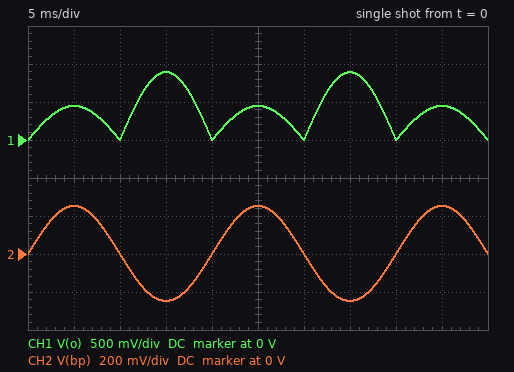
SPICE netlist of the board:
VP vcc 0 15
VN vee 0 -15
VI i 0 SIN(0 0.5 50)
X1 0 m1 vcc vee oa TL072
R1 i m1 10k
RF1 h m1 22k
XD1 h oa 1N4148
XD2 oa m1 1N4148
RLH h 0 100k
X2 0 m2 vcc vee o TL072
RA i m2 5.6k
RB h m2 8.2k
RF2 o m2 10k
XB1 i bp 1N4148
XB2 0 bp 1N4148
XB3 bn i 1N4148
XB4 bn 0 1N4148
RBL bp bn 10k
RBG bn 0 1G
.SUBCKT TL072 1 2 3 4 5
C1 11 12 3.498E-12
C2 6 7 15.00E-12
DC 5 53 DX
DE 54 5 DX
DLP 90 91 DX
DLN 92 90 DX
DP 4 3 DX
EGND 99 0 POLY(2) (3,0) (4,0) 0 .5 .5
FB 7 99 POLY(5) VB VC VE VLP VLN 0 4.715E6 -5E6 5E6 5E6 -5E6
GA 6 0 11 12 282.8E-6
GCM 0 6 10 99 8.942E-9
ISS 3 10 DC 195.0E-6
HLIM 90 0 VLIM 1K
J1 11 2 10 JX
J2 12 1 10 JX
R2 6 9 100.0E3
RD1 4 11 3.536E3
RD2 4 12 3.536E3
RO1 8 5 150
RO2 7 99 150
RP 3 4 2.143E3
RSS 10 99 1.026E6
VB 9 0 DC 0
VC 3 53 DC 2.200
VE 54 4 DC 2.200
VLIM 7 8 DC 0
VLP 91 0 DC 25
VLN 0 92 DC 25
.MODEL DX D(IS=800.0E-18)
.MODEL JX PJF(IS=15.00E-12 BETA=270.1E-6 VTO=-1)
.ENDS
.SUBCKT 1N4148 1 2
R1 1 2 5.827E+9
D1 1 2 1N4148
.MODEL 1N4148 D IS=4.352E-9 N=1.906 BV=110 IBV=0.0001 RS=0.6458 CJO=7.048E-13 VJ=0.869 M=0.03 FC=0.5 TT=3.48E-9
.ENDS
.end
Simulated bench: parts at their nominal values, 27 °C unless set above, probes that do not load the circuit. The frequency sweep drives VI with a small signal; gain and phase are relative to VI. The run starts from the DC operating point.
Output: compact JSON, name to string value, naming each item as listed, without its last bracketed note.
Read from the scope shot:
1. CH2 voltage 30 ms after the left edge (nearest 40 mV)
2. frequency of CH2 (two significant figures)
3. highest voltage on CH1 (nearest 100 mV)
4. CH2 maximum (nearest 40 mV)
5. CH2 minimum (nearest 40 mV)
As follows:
{"CH2 voltage 30 ms after the left edge": "0 V", "frequency of CH2": "50 Hz", "highest voltage on CH1": "900 mV", "CH2 maximum": "240 mV", "CH2 minimum": "-240 mV"}
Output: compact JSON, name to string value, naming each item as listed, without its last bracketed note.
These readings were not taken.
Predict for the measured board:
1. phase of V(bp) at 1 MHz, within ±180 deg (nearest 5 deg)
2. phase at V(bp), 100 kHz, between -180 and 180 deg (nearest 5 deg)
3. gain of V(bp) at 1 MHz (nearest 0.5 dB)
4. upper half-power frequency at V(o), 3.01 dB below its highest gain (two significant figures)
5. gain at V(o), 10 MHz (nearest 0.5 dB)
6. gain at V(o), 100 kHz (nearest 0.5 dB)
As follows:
{"phase of V(bp) at 1 MHz, within ±180 deg": "0 deg", "phase at V(bp), 100 kHz, between -180 and 180 deg": "0 deg", "gain of V(bp) at 1 MHz": "-6.0 dB", "upper half-power frequency at V(o), 3.01 dB below its highest gain": "1.3 MHz", "gain at V(o), 10 MHz": "-18.0 dB", "gain at V(o), 100 kHz": "5.5 dB"}
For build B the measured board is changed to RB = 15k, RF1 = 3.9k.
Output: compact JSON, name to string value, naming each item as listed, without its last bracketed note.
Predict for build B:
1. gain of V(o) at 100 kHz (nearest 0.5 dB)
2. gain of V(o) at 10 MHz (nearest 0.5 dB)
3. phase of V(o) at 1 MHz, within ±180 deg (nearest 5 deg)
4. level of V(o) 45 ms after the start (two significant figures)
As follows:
{"gain of V(o) at 100 kHz": "6.0 dB", "gain of V(o) at 10 MHz": "-17.5 dB", "phase of V(o) at 1 MHz, within ±180 deg": "130 deg", "level of V(o) 45 ms after the start": "-760 mV"}
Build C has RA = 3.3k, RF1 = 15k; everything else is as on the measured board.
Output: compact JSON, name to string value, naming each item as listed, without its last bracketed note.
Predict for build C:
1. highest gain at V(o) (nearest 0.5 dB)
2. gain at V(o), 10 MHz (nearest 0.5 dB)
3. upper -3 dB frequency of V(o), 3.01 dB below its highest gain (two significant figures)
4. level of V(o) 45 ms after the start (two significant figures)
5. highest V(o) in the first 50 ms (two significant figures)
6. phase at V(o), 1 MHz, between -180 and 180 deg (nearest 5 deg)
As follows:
{"highest gain at V(o)": "10.0 dB", "gain at V(o), 10 MHz": "-16.5 dB", "upper -3 dB frequency of V(o), 3.01 dB below its highest gain": "880 kHz", "level of V(o) 45 ms after the start": "-600 mV", "highest V(o) in the first 50 ms": "1.5 V", "phase at V(o), 1 MHz, between -180 and 180 deg": "120 deg"}
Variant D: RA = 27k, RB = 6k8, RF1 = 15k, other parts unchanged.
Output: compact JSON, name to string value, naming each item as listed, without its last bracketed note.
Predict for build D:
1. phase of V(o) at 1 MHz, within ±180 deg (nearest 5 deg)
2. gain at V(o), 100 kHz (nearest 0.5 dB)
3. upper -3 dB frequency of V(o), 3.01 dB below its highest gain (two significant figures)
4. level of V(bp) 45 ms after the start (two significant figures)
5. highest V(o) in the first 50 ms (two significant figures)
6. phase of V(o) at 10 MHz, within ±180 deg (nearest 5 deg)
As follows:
{"phase of V(o) at 1 MHz, within ±180 deg": "150 deg", "gain at V(o), 100 kHz": "-5.0 dB", "upper -3 dB frequency of V(o), 3.01 dB below its highest gain": "2.8 MHz", "level of V(bp) 45 ms after the start": "250 mV", "highest V(o) in the first 50 ms": "920 mV", "phase of V(o) at 10 MHz, within ±180 deg": "20 deg"}
